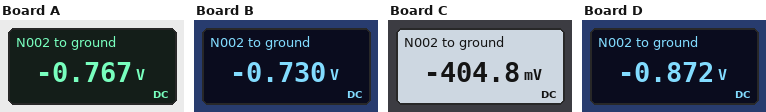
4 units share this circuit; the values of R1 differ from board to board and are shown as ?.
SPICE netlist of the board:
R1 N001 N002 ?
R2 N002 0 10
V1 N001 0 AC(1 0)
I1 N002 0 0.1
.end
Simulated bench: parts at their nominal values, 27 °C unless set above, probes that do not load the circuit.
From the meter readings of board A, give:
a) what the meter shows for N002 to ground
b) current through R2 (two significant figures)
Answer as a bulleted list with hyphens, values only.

- -0.767 V
- 77 mA
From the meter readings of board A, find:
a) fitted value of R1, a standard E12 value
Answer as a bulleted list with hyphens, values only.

- 33 Ω
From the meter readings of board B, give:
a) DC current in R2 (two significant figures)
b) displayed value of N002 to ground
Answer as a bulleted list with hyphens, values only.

- 73 mA
- -0.730 V
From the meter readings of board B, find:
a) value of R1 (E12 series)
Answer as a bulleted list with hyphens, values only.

- 27 Ω
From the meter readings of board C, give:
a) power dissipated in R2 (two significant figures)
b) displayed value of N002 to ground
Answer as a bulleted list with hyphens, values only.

- 16 mW
- -404.8 mV
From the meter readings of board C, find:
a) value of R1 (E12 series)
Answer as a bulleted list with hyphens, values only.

- 6.8 Ω
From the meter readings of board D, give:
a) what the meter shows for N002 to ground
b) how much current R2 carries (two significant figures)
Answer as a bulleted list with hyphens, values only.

- -0.872 V
- 87 mA
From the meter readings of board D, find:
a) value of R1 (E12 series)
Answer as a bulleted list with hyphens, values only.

- 68 Ω
